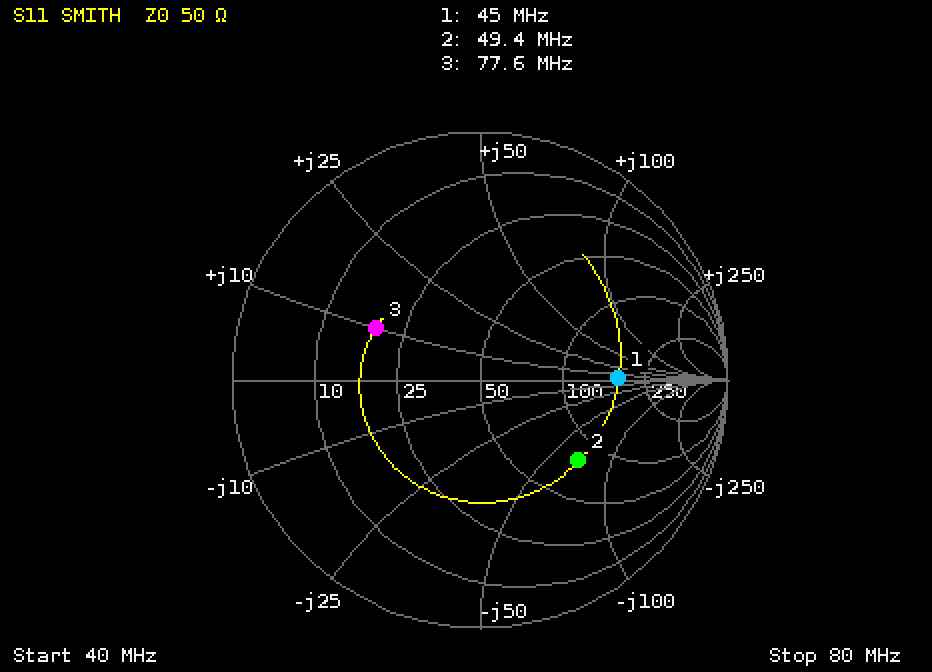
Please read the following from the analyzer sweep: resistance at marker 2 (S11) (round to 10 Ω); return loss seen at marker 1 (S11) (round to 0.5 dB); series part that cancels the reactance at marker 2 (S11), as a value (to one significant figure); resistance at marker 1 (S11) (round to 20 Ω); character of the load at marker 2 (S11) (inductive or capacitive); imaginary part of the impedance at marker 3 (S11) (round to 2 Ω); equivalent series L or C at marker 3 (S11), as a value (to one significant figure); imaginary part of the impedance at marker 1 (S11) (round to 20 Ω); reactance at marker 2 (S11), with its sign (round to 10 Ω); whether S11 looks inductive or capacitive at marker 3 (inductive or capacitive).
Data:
80 Ω
5.0 dB
200 nH
180 Ω
capacitive
+10 Ω
20 nH
0 Ω
-70 Ω
inductive
